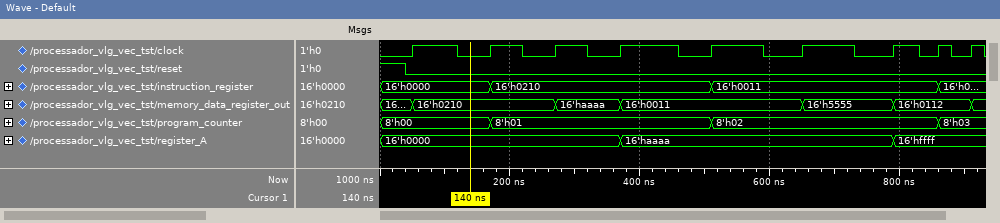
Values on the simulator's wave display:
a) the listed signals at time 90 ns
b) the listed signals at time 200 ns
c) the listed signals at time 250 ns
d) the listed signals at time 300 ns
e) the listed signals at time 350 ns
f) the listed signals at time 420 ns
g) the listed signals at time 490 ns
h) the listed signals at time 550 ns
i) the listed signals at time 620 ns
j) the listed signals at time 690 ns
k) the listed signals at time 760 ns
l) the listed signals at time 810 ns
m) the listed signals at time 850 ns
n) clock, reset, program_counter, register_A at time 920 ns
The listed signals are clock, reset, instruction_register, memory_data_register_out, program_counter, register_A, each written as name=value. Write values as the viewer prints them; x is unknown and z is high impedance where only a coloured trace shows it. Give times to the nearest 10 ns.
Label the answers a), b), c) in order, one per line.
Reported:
a) clock=1, reset=0, instruction_register=16'h0000, memory_data_register_out=16'h0210, program_counter=8'h00, register_A=16'h0000
b) clock=1, reset=0, instruction_register=16'h0210, memory_data_register_out=16'h0210, program_counter=8'h01, register_A=16'h0000
c) clock=0, reset=0, instruction_register=16'h0210, memory_data_register_out=16'h0210, program_counter=8'h01, register_A=16'h0000
d) clock=1, reset=0, instruction_register=16'h0210, memory_data_register_out=16'haaaa, program_counter=8'h01, register_A=16'h0000
e) clock=0, reset=0, instruction_register=16'h0210, memory_data_register_out=16'haaaa, program_counter=8'h01, register_A=16'h0000
f) clock=1, reset=0, instruction_register=16'h0210, memory_data_register_out=16'h0011, program_counter=8'h01, register_A=16'haaaa
g) clock=0, reset=0, instruction_register=16'h0210, memory_data_register_out=16'h0011, program_counter=8'h01, register_A=16'haaaa
h) clock=1, reset=0, instruction_register=16'h0011, memory_data_register_out=16'h0011, program_counter=8'h02, register_A=16'haaaa
i) clock=0, reset=0, instruction_register=16'h0011, memory_data_register_out=16'h0011, program_counter=8'h02, register_A=16'haaaa
j) clock=1, reset=0, instruction_register=16'h0011, memory_data_register_out=16'h5555, program_counter=8'h02, register_A=16'haaaa
k) clock=0, reset=0, instruction_register=16'h0011, memory_data_register_out=16'h5555, program_counter=8'h02, register_A=16'haaaa
l) clock=1, reset=0, instruction_register=16'h0011, memory_data_register_out=16'h0112, program_counter=8'h02, register_A=16'hffff
m) clock=0, reset=0, instruction_register=16'h0011, memory_data_register_out=16'h0112, program_counter=8'h02, register_A=16'hffff
n) clock=1, reset=0, program_counter=8'h03, register_A=16'hffff
